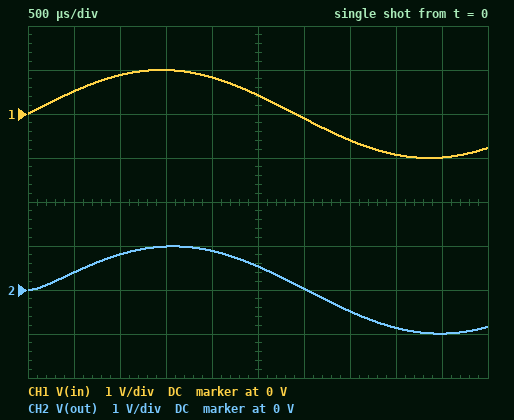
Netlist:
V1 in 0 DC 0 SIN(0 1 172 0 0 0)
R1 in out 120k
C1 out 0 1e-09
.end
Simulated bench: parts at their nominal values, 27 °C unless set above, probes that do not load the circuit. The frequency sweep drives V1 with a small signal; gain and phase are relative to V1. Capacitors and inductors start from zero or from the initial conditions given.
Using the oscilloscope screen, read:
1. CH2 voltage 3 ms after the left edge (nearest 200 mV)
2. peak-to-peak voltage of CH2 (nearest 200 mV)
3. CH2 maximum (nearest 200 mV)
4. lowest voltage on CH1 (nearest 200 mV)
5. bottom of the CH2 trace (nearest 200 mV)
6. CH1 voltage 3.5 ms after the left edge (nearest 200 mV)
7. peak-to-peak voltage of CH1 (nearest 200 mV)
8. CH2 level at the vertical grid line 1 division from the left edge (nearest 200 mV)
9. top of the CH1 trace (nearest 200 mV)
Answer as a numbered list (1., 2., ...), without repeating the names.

1. 0 V
2. 2.0 V
3. 1.0 V
4. -1.0 V
5. -1.0 V
6. -600 mV
7. 2.0 V
8. 400 mV
9. 1.0 V
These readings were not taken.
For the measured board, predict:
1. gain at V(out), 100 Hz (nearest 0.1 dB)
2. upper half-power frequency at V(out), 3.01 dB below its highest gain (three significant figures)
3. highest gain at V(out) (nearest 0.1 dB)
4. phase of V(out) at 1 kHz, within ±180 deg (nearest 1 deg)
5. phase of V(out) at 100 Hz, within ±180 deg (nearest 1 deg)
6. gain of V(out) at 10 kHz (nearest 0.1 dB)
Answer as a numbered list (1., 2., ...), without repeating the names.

1. 0 dB
2. 1.33 kHz
3. 0 dB
4. -37 deg
5. -4 deg
6. -17.6 dB
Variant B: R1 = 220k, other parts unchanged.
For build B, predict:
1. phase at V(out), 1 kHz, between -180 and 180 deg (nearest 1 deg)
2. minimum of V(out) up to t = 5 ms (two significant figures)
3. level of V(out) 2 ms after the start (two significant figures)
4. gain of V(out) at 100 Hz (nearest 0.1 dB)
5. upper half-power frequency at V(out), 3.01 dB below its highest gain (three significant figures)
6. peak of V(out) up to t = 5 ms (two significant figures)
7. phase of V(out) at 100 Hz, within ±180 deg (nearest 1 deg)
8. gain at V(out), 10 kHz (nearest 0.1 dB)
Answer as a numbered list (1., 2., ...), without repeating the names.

1. -54 deg
2. -970 mV
3. 910 mV
4. -0.1 dB
5. 723 Hz
6. 970 mV
7. -8 deg
8. -22.8 dB
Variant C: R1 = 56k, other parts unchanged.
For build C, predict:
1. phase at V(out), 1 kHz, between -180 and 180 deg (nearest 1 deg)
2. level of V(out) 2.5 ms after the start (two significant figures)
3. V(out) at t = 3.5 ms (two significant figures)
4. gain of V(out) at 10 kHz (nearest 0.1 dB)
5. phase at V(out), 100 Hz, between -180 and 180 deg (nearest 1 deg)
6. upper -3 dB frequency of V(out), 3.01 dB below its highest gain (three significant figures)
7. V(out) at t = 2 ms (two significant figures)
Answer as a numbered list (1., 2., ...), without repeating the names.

1. -19 deg
2. 480 mV
3. -550 mV
4. -11.3 dB
5. -2 deg
6. 2.84 kHz
7. 860 mV
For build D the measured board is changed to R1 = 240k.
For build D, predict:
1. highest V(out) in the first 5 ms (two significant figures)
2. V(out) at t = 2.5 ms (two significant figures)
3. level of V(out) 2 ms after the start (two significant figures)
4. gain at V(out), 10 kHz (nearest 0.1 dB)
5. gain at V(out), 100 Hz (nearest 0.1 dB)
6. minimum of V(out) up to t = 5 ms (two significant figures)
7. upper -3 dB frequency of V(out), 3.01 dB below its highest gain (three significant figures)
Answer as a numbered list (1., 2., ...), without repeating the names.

1. 970 mV
2. 620 mV
3. 910 mV
4. -23.6 dB
5. -0.1 dB
6. -970 mV
7. 663 Hz
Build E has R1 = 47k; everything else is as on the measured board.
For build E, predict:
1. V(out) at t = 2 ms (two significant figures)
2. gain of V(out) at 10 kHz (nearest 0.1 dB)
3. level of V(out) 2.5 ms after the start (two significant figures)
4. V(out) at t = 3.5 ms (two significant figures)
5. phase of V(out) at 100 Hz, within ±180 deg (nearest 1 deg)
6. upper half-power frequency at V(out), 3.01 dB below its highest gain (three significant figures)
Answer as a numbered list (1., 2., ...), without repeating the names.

1. 860 mV
2. -9.9 dB
3. 470 mV
4. -560 mV
5. -2 deg
6. 3.39 kHz
